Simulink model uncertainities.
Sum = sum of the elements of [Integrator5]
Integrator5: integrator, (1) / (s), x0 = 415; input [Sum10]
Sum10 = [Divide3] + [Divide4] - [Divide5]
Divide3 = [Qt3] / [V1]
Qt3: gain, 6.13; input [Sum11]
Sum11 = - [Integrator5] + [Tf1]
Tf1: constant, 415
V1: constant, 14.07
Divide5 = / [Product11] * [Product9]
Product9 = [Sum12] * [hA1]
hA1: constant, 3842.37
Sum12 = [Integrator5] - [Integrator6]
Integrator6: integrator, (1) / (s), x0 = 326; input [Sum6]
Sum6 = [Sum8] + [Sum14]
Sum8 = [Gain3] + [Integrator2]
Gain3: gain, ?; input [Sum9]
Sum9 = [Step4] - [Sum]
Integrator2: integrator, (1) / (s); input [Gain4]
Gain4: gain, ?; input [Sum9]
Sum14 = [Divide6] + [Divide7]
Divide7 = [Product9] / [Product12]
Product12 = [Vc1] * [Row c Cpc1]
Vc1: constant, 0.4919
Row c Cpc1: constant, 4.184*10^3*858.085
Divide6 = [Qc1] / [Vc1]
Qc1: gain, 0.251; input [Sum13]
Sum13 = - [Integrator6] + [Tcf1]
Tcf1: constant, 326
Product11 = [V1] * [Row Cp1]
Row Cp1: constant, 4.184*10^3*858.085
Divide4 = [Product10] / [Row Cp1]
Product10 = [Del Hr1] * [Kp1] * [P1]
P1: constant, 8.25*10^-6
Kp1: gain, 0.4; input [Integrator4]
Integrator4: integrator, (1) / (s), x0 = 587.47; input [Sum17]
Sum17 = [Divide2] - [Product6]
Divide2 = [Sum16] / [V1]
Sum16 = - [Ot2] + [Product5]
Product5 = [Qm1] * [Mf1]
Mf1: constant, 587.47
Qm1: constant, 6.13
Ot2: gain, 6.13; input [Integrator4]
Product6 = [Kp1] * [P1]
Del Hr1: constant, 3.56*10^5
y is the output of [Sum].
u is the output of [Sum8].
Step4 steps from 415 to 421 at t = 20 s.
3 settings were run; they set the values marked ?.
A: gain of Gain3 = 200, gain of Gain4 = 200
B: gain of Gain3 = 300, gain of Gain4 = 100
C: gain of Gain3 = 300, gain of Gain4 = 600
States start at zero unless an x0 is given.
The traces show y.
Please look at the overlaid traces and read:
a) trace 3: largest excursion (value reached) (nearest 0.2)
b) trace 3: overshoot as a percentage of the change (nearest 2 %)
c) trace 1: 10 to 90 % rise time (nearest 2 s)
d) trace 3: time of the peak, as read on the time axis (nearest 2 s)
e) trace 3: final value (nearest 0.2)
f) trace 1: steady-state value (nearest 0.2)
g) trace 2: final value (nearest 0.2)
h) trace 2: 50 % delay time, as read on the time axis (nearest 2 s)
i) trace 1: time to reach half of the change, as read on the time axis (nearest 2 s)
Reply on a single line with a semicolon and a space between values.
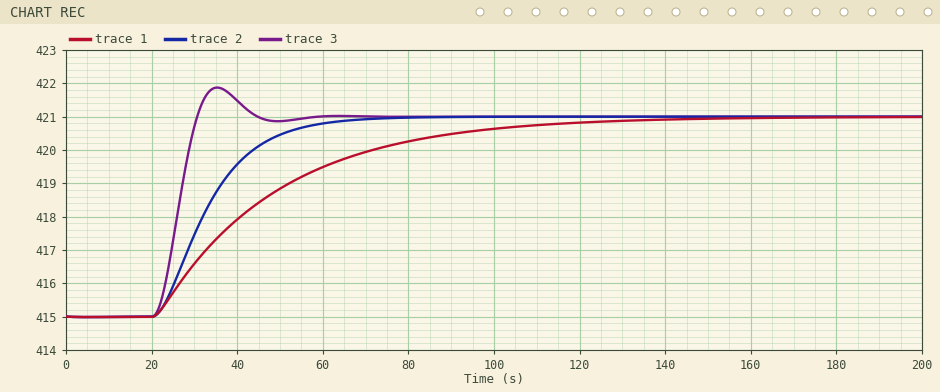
421.8; 14 %; 62 s; 36 s; 421.0; 421.0; 421.0; 32 s; 40 s
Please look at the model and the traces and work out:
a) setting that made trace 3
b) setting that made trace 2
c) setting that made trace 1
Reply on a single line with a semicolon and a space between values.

C; A; B
